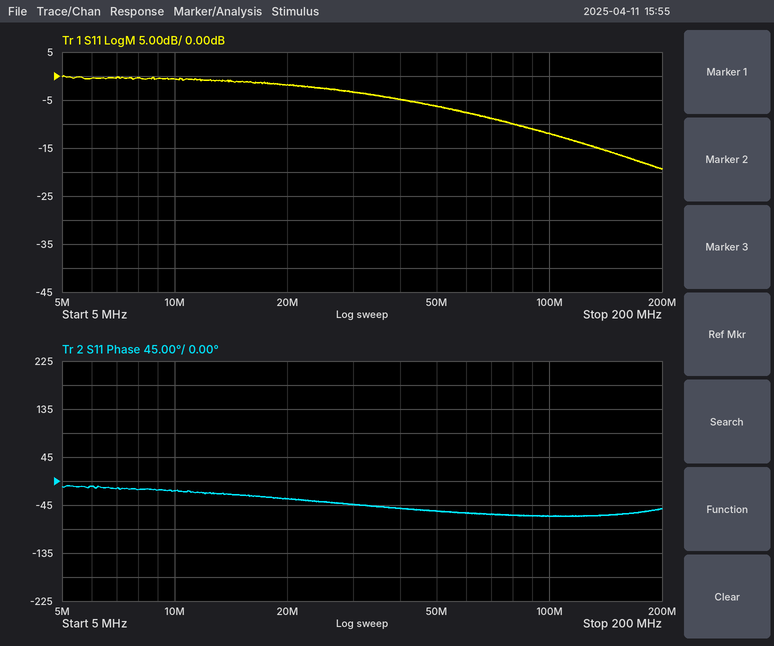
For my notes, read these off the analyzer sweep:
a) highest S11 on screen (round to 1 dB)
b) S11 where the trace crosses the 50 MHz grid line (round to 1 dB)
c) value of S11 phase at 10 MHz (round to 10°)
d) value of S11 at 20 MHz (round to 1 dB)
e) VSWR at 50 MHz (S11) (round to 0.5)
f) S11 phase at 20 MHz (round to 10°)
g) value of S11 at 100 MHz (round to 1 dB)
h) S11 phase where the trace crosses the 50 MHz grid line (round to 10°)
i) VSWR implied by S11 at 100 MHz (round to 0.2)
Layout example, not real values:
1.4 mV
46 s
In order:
0 dB
-6 dB
-20°
-2 dB
3.0
-30°
-12 dB
-60°
1.6
